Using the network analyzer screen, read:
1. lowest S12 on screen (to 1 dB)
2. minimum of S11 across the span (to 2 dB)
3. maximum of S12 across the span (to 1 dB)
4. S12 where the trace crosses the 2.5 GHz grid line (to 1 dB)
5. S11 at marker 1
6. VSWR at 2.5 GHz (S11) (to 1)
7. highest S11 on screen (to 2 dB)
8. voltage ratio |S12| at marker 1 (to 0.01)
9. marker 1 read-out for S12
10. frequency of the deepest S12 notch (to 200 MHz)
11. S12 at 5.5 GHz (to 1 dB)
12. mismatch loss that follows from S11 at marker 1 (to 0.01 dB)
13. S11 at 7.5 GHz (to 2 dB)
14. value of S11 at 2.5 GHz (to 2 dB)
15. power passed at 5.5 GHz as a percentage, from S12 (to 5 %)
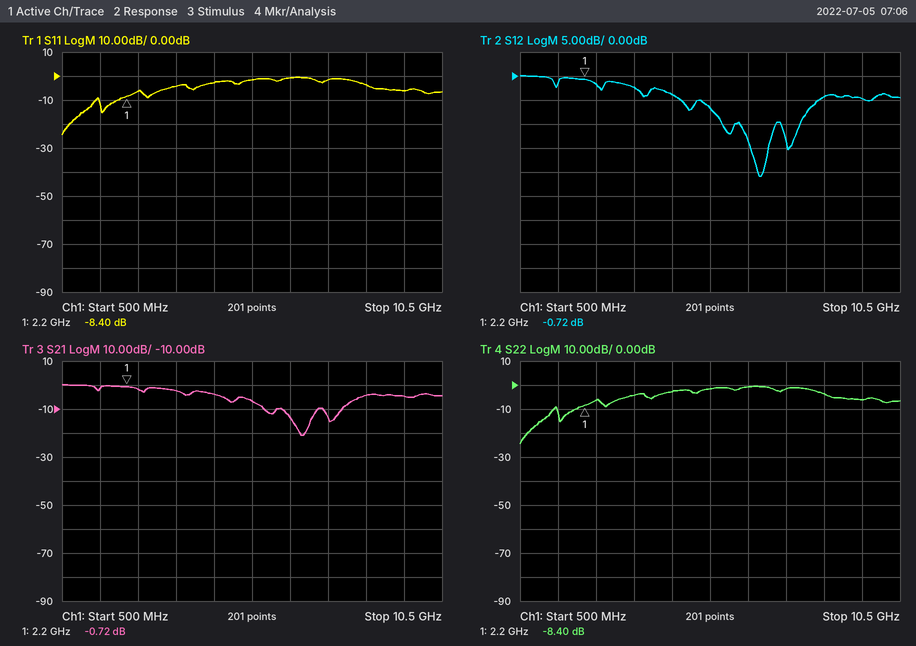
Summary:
-21 dB
-24 dB
0 dB
-2 dB
-8.40 dB
3
0 dB
0.92
-0.72 dB
6.8 GHz
-7 dB
0.68 dB
-2 dB
-6 dB
20 %
